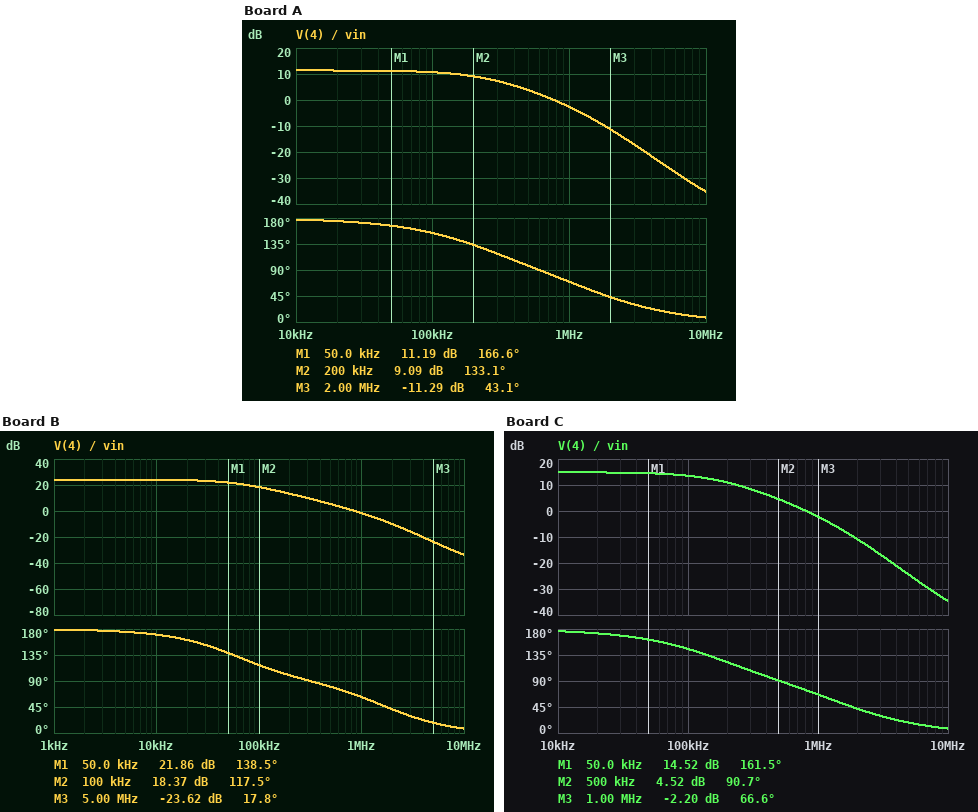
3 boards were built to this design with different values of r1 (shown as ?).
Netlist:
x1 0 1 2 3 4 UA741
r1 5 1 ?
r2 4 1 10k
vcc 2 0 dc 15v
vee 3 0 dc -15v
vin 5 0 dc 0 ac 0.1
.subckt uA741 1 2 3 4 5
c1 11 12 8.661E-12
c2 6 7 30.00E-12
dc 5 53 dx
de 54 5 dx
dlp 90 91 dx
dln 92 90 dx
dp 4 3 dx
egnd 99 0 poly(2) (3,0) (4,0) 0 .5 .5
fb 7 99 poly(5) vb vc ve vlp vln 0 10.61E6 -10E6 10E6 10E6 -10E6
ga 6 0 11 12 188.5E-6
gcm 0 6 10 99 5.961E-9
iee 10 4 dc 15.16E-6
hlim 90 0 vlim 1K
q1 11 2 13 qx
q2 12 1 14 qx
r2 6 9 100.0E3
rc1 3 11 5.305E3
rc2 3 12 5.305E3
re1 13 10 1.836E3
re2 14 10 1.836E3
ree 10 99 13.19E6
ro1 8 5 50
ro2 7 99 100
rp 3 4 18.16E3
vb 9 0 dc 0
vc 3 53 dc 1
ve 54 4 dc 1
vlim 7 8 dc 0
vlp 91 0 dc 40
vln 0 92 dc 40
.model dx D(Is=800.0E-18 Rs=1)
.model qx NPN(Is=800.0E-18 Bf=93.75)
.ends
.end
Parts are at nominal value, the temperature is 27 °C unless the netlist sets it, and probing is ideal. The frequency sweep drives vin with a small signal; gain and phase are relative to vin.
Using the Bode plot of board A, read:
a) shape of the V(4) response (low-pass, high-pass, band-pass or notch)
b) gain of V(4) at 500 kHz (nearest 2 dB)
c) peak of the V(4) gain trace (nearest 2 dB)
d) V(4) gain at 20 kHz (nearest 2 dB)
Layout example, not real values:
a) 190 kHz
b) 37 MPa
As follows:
a) low-pass
b) 4 dB
c) 12 dB
d) 12 dB
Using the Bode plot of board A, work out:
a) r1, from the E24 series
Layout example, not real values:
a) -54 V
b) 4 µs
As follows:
a) 2.7 kΩ
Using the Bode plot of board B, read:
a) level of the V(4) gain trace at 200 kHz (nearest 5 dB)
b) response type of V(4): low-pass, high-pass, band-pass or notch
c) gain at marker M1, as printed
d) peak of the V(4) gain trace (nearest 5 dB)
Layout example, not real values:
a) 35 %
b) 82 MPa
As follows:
a) 15 dB
b) low-pass
c) 21.86 dB
d) 25 dB
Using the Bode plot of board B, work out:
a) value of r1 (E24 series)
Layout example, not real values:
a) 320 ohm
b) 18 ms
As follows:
a) 620 Ω
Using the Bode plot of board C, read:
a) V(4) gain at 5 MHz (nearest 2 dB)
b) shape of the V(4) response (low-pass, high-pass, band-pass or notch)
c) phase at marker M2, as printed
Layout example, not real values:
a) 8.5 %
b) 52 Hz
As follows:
a) -24 dB
b) low-pass
c) 90.7 deg
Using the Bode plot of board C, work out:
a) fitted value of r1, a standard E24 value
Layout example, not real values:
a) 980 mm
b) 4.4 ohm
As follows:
a) 1.8 kΩ
